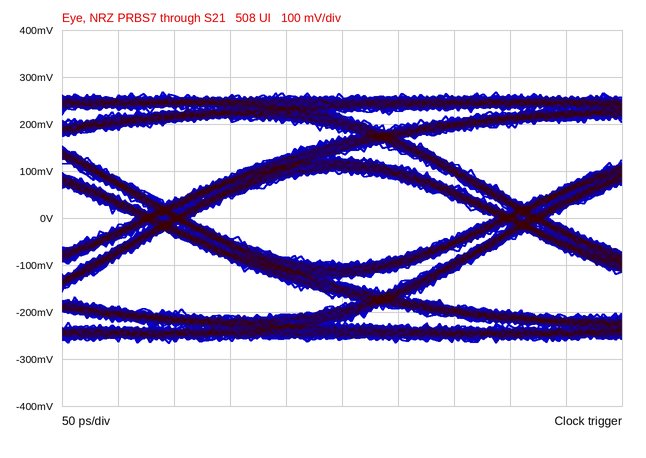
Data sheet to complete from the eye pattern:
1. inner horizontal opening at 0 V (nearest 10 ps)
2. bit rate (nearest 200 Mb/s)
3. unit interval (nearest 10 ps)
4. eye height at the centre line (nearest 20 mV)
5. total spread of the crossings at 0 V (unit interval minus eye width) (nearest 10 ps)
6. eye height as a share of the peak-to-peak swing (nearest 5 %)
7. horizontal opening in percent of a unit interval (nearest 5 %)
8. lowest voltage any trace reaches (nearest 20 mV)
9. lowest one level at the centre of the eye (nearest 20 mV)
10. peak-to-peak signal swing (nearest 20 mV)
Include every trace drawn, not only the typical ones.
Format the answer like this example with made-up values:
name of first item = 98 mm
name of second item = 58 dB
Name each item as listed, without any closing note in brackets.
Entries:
inner horizontal opening at 0 V = 270 ps
bit rate = 3.2 Gb/s
unit interval = 320 ps
eye height at the centre line = 200 mV
total spread of the crossings at 0 V (unit interval minus eye width) = 50 ps
eye height as a share of the peak-to-peak swing = 35 %
horizontal opening in percent of a unit interval = 85 %
lowest voltage any trace reaches = -260 mV
lowest one level at the centre of the eye = 100 mV
peak-to-peak signal swing = 540 mV
